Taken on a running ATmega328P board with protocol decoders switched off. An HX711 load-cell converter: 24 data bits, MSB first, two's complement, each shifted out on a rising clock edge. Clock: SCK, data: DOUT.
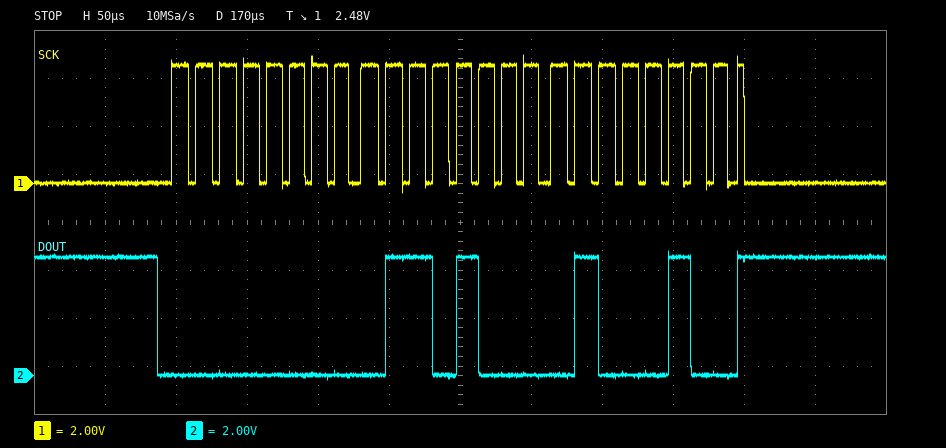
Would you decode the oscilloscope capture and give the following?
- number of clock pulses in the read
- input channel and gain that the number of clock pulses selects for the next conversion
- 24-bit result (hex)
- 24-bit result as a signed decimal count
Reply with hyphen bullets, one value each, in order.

- 25
- channel A, gain 128
- 0x006844
- 26692
